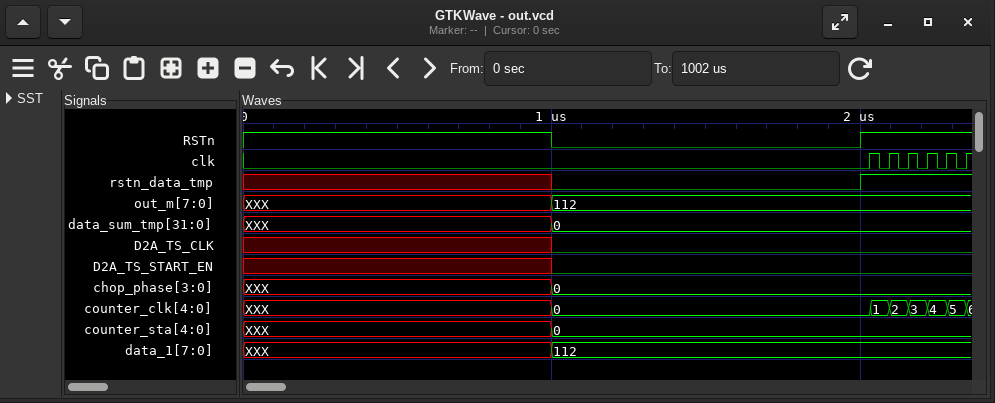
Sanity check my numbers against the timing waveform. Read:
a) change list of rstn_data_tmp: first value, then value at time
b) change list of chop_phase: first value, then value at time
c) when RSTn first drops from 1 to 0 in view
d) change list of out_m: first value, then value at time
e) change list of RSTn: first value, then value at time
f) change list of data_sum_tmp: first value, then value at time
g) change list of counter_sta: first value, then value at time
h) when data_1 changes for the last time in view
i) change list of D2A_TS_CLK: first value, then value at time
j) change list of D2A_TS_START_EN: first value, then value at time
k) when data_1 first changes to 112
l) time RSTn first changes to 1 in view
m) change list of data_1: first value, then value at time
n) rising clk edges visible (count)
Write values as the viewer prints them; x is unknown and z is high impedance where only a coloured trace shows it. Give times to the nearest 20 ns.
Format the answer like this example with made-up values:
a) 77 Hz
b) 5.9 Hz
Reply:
a) x, 0 at 1000 ns, 1 at 2000 ns
b) XXX, 0 at 1000 ns
c) 1000 ns
d) XXX, 112 at 1000 ns
e) 1, 0 at 1000 ns, 1 at 2000 ns
f) XXX, 0 at 1000 ns
g) XXX, 0 at 1000 ns
h) 1000 ns
i) x, 0 at 1000 ns
j) x, 0 at 1000 ns
k) 1000 ns
l) 2000 ns
m) XXX, 112 at 1000 ns
n) 6
